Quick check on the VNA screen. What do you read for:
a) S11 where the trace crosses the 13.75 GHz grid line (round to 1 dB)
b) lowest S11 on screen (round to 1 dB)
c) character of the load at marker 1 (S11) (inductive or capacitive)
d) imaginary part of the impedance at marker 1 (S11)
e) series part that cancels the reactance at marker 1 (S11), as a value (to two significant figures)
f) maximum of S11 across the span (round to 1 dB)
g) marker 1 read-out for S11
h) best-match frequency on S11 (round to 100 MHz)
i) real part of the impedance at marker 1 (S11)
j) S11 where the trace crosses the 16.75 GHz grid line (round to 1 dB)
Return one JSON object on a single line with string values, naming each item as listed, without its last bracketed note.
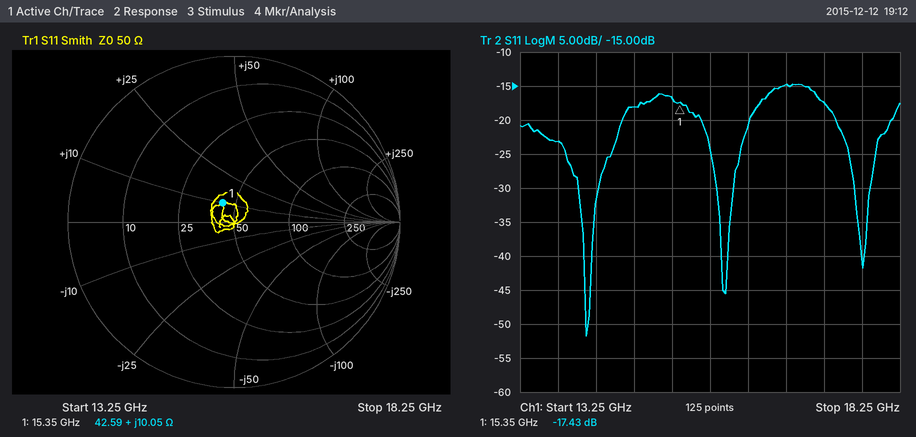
{"S11 where the trace crosses the 13.75 GHz grid line": "-23 dB", "lowest S11 on screen": "-52 dB", "character of the load at marker 1 (S11)": "inductive", "imaginary part of the impedance at marker 1": "+10.05 Ω", "series part that cancels the reactance at marker 1 (S11), as a value": "1.0 pF", "maximum of S11 across the span": "-15 dB", "marker 1 read-out for S11": "-17.43 dB", "best-match frequency on S11": "14.1 GHz", "real part of the impedance at marker 1": "42.59 Ω", "S11 where the trace crosses the 16.75 GHz grid line": "-15 dB"}
